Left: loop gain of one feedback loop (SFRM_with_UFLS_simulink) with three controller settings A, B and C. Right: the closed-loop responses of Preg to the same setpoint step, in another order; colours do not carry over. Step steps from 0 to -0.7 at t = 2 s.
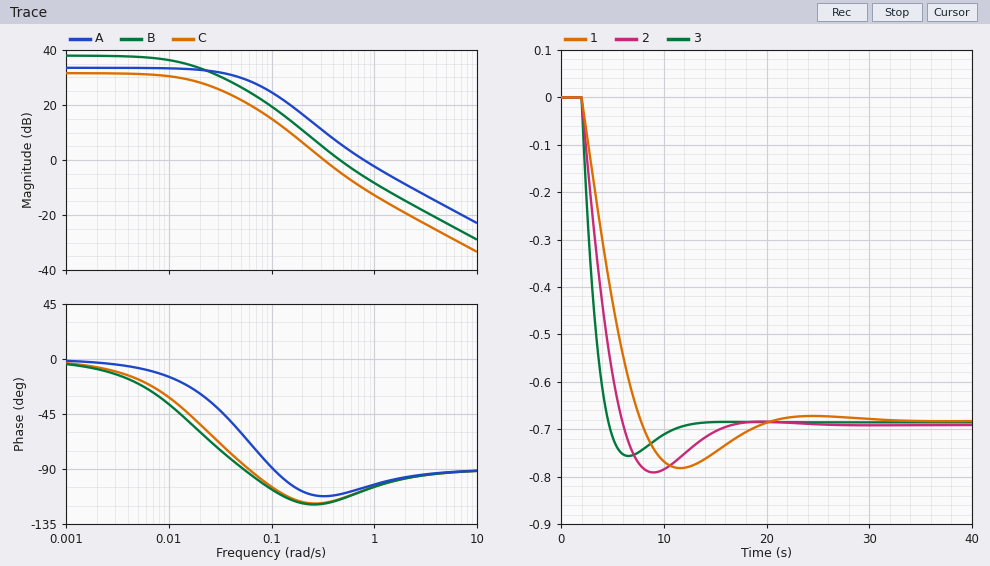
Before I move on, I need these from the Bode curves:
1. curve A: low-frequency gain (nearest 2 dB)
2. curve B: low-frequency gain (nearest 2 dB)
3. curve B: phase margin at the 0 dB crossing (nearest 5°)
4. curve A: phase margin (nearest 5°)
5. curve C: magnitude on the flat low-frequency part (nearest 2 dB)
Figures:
34 dB
38 dB
65°
75°
32 dB
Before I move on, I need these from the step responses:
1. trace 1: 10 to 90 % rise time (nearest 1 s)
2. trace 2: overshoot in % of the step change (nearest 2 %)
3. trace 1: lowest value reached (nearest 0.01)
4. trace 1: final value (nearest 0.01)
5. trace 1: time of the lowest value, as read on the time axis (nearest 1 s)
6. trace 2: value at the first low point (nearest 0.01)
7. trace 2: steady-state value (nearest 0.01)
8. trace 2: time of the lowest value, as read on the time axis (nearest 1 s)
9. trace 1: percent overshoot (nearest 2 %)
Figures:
4 s
14 %
-0.78
-0.68
12 s
-0.79
-0.69
9 s
14 %
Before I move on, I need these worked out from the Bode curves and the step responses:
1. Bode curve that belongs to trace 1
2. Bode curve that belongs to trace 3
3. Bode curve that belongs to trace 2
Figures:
C
A
B
